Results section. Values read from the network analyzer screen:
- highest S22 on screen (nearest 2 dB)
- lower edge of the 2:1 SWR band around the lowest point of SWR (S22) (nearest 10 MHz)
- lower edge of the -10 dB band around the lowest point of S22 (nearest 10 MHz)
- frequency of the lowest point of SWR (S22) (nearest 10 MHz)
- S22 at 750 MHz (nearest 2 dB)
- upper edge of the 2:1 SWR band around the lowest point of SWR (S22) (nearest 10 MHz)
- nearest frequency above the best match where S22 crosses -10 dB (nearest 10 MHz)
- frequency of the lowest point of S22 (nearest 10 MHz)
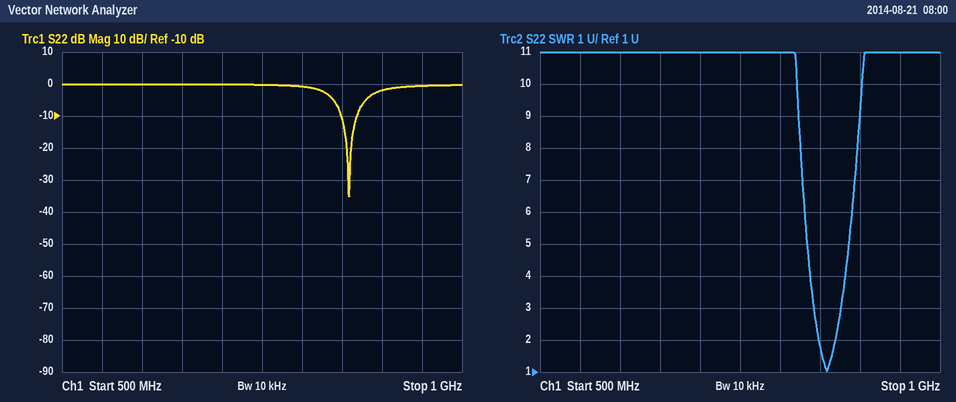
0 dB
850 MHz
850 MHz
860 MHz
0 dB
870 MHz
870 MHz
860 MHz
